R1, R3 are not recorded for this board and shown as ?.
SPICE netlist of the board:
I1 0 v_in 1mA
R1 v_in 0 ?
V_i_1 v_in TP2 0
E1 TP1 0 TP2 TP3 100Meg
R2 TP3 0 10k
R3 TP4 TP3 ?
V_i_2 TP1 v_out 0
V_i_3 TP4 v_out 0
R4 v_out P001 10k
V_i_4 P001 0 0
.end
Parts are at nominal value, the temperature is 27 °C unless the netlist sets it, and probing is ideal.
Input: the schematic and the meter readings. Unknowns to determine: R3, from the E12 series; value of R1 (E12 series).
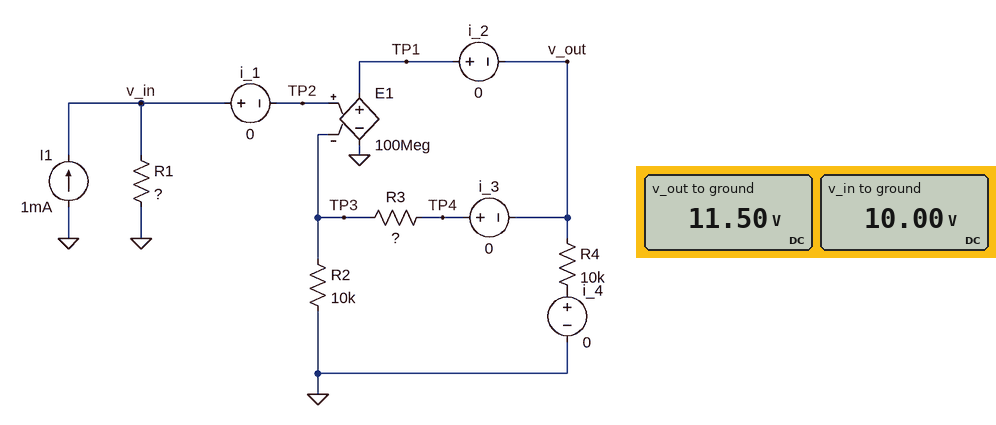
1.5 kΩ
10 kΩ
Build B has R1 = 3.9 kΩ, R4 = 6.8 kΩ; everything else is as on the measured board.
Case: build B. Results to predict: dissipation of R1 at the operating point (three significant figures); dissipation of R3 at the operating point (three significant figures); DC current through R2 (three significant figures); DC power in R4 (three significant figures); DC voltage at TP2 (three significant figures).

3.90 mW
228 µW
390 µA
2.96 mW
3.90 V
